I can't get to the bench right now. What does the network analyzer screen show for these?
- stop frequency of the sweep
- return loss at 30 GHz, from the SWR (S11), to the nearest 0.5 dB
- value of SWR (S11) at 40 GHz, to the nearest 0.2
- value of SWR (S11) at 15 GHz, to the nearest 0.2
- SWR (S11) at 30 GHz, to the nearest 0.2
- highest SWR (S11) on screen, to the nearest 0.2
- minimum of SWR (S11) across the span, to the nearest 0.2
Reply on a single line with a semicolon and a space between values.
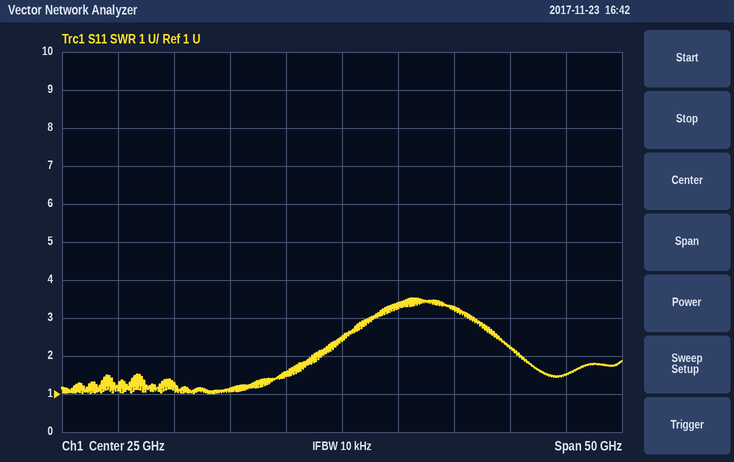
50 GHz; 5.5 dB; 2.2; 1.2; 3.4; 3.6; 1.0
